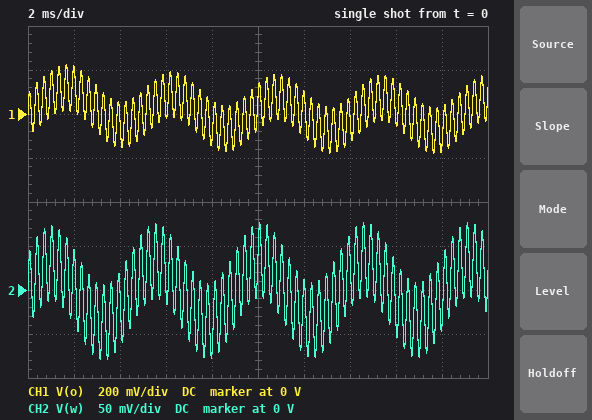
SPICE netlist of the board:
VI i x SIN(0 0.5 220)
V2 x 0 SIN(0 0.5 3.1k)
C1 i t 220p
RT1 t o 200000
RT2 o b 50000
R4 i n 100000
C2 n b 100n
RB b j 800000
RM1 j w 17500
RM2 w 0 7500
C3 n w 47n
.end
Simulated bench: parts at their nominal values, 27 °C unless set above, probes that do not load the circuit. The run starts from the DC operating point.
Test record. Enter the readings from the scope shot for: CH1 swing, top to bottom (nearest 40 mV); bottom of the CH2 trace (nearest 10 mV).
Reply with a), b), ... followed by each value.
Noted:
a) 400 mV
b) -80 mV
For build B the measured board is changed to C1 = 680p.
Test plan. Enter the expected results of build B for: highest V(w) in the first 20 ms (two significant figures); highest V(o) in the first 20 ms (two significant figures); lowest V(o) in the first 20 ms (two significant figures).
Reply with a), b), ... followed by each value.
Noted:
a) 81 mV
b) 250 mV
c) -200 mV
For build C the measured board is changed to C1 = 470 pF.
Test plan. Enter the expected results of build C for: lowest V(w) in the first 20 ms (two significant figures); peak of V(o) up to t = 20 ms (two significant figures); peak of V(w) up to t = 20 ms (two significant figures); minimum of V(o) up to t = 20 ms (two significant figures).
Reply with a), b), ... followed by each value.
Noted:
a) -82 mV
b) 240 mV
c) 80 mV
d) -200 mV
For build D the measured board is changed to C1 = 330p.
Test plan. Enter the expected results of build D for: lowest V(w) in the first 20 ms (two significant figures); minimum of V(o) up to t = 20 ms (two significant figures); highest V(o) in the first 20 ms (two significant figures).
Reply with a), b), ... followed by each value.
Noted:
a) -81 mV
b) -190 mV
c) 240 mV
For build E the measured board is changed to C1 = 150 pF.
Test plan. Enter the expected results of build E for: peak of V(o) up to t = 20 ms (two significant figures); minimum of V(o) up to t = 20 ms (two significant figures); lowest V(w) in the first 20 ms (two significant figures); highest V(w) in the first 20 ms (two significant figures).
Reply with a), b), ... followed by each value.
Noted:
a) 210 mV
b) -160 mV
c) -76 mV
d) 74 mV
